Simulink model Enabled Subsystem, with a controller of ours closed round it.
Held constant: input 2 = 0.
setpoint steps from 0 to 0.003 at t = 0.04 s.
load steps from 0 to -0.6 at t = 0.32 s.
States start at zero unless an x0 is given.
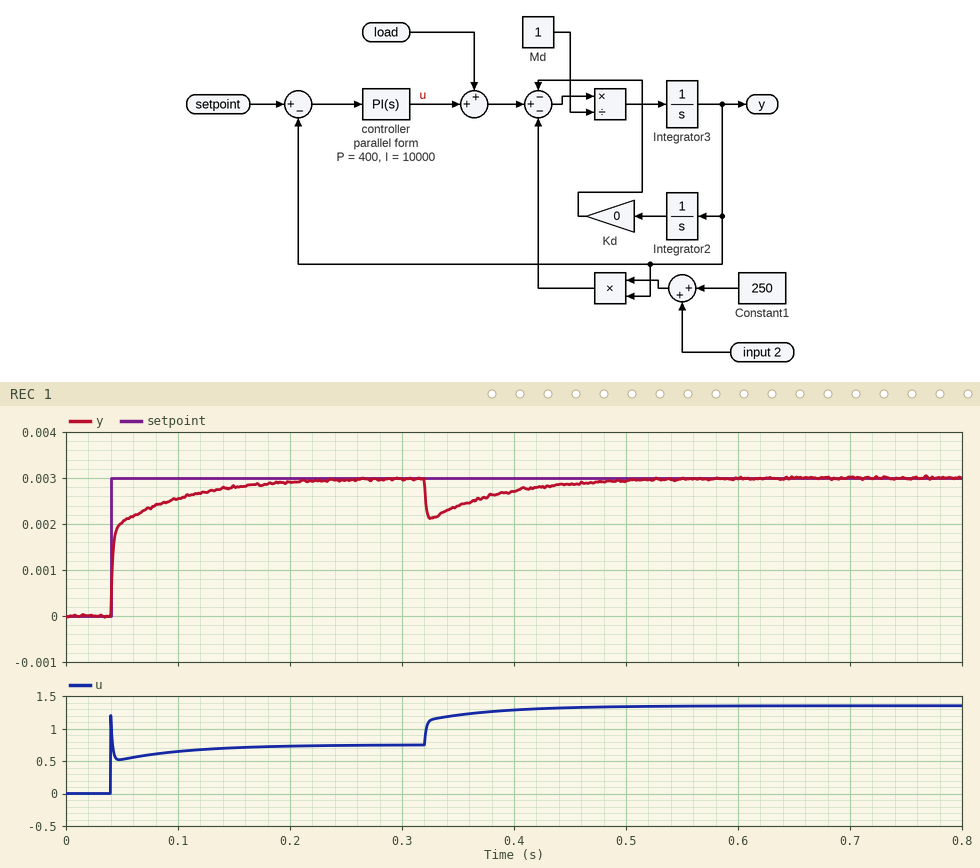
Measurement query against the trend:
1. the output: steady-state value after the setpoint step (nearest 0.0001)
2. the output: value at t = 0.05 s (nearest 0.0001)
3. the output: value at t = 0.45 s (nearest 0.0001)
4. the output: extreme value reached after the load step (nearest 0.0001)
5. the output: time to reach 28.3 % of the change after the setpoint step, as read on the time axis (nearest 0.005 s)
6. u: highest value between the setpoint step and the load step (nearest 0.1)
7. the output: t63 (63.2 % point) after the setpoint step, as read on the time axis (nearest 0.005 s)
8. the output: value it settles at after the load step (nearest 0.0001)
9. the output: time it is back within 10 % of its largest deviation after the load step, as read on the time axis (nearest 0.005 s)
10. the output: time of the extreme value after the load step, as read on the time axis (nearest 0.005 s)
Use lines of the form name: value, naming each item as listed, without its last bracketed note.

the output: steady-state value after the setpoint step: 0.0030
the output: value at t = 0.05 s: 0.0020
the output: value at t = 0.45 s: 0.0029
the output: extreme value reached after the load step: 0.0021
the output: time to reach 28.3 % of the change after the setpoint step, as read on the time axis: 0.040 s
u: highest value between the setpoint step and the load step: 1.2
the output: t63 (63.2 % point) after the setpoint step, as read on the time axis: 0.045 s
the output: value it settles at after the load step: 0.0030
the output: time it is back within 10 % of its largest deviation after the load step, as read on the time axis: 0.475 s
the output: time of the extreme value after the load step, as read on the time axis: 0.325 s
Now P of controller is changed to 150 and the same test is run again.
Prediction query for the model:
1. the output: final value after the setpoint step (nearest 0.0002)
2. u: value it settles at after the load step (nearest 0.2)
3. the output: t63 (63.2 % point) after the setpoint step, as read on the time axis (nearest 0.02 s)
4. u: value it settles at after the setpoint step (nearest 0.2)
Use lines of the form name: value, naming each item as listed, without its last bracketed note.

the output: final value after the setpoint step: 0.0030
u: value it settles at after the load step: 1.4
the output: t63 (63.2 % point) after the setpoint step, as read on the time axis: 0.06 s
u: value it settles at after the setpoint step: 0.8
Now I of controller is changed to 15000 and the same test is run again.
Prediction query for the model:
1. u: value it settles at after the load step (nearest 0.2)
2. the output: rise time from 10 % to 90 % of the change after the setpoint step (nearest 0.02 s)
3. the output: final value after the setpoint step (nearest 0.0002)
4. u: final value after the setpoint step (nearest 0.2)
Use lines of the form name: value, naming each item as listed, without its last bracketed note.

u: value it settles at after the load step: 1.4
the output: rise time from 10 % to 90 % of the change after the setpoint step: 0.06 s
the output: final value after the setpoint step: 0.0030
u: final value after the setpoint step: 0.8
